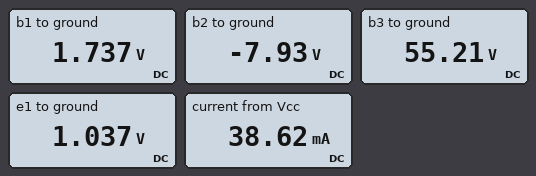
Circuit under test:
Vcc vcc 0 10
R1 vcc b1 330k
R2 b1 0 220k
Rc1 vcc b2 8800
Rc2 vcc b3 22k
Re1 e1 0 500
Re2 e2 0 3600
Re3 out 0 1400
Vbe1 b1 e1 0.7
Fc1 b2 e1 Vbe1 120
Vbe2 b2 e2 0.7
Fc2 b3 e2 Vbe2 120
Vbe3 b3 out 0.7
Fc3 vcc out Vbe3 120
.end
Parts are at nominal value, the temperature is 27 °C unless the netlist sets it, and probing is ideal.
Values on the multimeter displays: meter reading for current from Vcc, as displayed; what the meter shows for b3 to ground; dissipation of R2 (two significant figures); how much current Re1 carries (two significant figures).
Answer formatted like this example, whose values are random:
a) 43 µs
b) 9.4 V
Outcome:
a) 38.62 mA
b) 55.21 V
c) 14 µW
d) 2.1 mA
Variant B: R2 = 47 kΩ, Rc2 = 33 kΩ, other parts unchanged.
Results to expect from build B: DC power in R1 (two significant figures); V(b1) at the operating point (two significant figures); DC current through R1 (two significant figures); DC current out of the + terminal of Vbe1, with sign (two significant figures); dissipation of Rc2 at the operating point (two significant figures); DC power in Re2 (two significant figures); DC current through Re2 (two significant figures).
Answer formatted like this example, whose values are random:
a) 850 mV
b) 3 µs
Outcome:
a) 240 µW
b) 1.0 V
c) 27 µA
d) -5.4 µA
e) 25 mW
f) 3.5 mW
g) 990 µA
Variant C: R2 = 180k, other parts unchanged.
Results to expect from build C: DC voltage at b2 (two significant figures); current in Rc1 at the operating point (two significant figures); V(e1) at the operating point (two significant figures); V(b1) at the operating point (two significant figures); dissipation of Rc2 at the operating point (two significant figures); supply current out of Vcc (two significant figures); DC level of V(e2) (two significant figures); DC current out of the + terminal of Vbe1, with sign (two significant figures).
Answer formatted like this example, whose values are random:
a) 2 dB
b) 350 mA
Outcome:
a) -6.7 V
b) 1.9 mA
c) 970 mV
d) 1.7 V
e) 68 mW
f) 34 mA
g) -7.4 V
h) -16 µA
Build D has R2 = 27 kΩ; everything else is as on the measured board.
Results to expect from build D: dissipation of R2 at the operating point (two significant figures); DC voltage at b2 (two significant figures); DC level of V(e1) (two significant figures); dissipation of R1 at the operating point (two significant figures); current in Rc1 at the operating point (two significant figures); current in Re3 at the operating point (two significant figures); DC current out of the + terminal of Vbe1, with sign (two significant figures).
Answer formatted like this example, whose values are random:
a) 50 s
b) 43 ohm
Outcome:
a) 20 µW
b) 9.1 V
c) 40 mV
d) 260 µW
e) 98 µA
f) 26 mA
g) -660 nA
